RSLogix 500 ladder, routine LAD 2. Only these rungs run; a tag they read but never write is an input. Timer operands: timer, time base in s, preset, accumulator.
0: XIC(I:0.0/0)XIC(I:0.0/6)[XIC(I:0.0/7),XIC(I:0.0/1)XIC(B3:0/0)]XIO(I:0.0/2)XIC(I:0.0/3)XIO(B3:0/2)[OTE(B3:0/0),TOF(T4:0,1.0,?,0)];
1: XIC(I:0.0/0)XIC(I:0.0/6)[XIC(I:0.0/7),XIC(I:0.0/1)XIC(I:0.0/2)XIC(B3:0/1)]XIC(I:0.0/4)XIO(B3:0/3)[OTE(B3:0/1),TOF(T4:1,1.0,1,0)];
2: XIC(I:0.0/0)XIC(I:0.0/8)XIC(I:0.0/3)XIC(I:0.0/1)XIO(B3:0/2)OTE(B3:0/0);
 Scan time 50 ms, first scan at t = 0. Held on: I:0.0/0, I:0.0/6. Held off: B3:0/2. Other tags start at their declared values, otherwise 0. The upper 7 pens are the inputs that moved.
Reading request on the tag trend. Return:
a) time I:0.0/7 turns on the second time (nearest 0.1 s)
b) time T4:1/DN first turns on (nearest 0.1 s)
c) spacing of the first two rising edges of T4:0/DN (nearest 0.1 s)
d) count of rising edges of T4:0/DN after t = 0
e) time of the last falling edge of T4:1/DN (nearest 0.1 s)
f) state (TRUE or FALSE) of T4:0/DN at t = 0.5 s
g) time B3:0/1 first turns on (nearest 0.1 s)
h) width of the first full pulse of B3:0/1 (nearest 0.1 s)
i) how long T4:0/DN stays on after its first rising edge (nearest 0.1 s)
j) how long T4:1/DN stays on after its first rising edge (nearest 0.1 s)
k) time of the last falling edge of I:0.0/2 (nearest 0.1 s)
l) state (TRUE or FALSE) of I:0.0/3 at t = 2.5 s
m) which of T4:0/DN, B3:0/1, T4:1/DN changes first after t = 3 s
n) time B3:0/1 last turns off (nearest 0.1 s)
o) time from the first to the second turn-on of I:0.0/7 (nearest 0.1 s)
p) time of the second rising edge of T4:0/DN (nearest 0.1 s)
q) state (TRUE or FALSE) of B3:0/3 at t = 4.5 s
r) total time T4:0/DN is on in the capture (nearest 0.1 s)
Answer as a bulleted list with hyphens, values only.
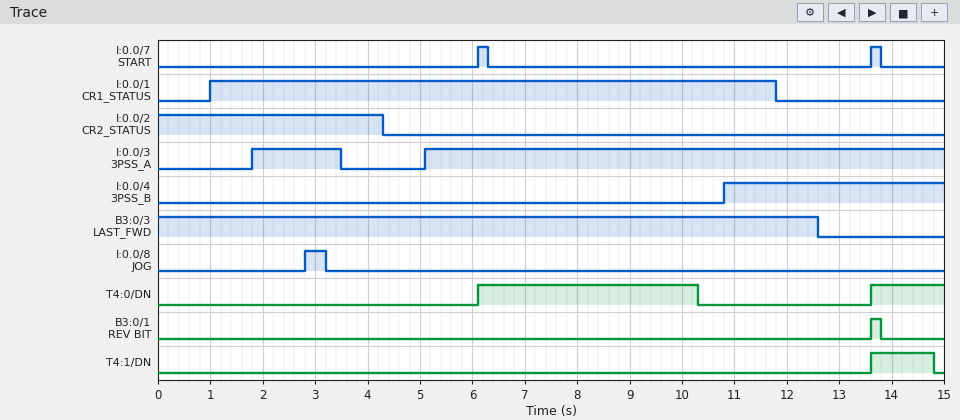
- 13.6 s
- 13.6 s
- 7.5 s
- 2
- 14.8 s
- FALSE
- 13.6 s
- 0.2 s
- 4.2 s
- 1.2 s
- 4.3 s
- TRUE
- T4:0/DN
- 13.8 s
- 7.5 s
- 13.6 s
- TRUE
- 5.6 s
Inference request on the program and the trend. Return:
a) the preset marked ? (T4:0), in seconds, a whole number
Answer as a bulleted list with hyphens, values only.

- 4 s
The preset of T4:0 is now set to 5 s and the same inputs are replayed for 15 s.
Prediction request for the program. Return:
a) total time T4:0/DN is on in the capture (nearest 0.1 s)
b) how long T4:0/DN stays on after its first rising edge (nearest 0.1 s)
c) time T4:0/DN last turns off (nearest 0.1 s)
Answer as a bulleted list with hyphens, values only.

- 6.6 s
- 5.2 s
- 11.3 s
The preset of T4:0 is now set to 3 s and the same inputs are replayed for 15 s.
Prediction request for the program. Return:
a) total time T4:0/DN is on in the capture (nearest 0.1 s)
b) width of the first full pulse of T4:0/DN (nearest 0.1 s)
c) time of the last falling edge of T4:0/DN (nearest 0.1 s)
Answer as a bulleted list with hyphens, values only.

- 4.6 s
- 3.2 s
- 9.3 s
